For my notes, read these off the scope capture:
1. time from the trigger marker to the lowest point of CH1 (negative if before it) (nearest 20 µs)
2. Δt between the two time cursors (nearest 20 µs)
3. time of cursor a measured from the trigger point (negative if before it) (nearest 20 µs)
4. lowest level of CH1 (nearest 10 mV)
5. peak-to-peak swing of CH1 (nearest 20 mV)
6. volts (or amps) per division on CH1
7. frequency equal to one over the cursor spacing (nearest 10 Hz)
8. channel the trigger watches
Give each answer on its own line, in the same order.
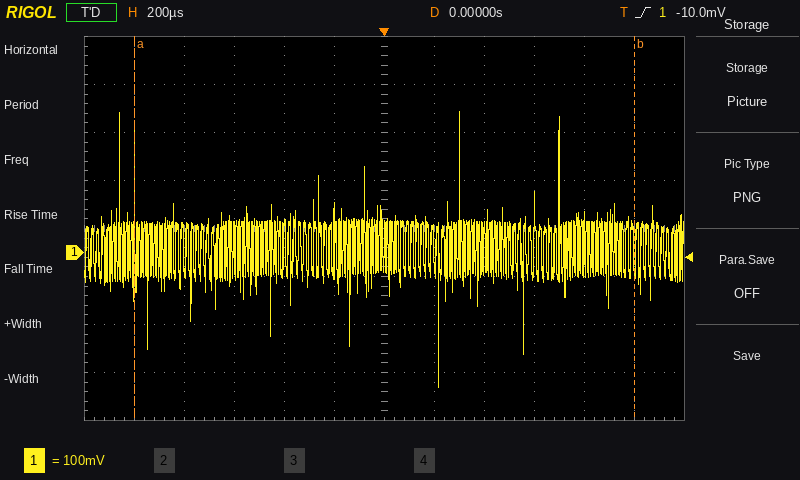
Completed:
+220 µs
2.00 ms
-1.00 ms
-280 mV
580 mV
100 mV
500 Hz
CH1
